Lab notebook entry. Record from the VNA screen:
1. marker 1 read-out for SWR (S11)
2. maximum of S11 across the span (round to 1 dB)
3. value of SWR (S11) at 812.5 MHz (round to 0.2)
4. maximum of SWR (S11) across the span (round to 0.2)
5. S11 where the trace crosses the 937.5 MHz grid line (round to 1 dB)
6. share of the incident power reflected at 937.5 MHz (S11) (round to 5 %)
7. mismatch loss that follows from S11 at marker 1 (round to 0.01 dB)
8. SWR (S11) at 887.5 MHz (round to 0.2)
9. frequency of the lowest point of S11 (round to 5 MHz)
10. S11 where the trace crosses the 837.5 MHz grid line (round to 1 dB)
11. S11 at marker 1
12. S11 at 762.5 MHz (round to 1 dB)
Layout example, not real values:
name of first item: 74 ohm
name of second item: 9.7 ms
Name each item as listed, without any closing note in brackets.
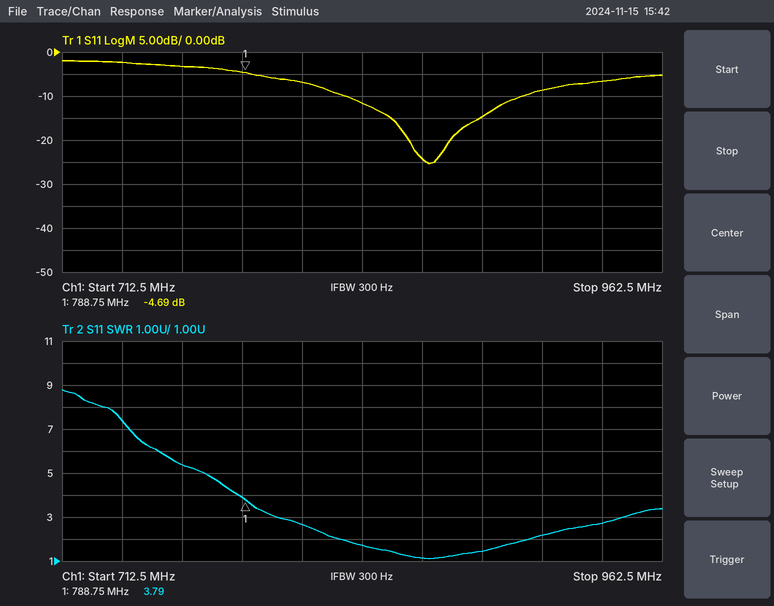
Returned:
marker 1 read-out for SWR: 3.79
maximum of S11 across the span: -2 dB
value of SWR (S11) at 812.5 MHz: 2.6
maximum of SWR (S11) across the span: 8.8
S11 where the trace crosses the 937.5 MHz grid line: -7 dB
share of the incident power reflected at 937.5 MHz (S11): 20 %
mismatch loss that follows from S11 at marker 1: 1.80 dB
SWR (S11) at 887.5 MHz: 1.4
frequency of the lowest point of S11: 865 MHz
S11 where the trace crosses the 837.5 MHz grid line: -12 dB
S11 at marker 1: -4.69 dB
S11 at 762.5 MHz: -3 dB
